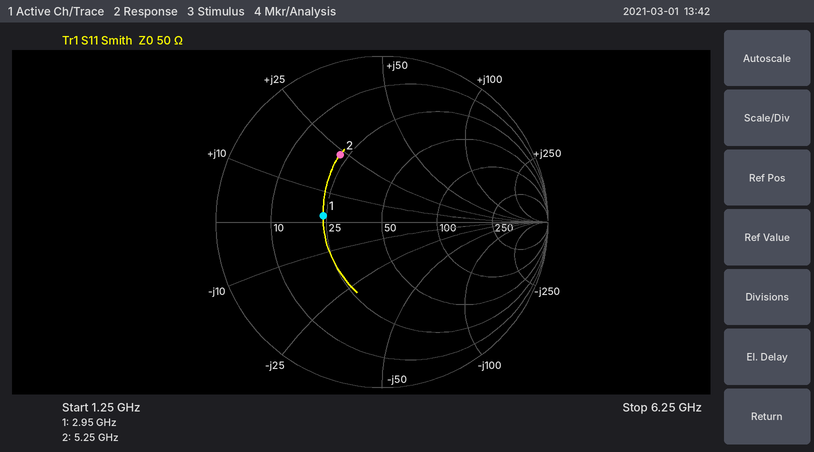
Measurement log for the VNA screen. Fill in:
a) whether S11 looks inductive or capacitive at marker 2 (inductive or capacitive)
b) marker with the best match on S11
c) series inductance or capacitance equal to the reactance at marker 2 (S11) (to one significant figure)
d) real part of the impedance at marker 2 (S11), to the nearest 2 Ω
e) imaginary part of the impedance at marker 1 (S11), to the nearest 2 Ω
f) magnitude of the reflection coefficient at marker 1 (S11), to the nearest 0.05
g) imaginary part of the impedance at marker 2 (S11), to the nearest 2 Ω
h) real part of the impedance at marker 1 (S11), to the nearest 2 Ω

inductive
marker 1
700 pH
22 Ω
+2 Ω
0.35
+24 Ω
24 Ω
